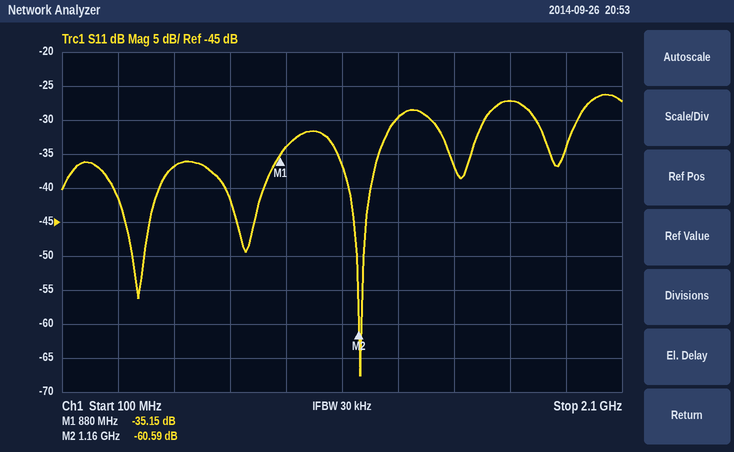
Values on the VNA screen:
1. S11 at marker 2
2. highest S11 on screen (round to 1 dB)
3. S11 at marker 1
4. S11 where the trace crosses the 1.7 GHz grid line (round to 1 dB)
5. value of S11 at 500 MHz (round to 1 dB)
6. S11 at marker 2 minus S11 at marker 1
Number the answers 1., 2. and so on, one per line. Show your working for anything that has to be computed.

1. -60.59 dB
2. -26 dB
3. -35.15 dB
4. -27 dB
5. -37 dB
6. -60.59 − (-35.15) = -25.44 dB
